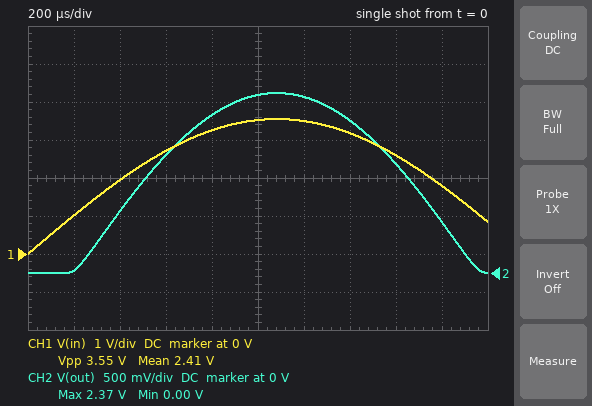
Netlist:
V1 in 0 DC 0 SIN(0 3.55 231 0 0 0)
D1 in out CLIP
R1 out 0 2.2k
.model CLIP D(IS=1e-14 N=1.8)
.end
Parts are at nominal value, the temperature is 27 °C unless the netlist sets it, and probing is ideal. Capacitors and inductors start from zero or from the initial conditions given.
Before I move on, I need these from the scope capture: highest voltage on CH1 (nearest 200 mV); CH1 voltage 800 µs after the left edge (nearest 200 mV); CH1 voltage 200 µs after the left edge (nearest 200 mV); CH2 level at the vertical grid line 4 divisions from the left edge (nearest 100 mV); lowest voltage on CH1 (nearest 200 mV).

3.6 V
3.2 V
1.0 V
2.1 V
0 V
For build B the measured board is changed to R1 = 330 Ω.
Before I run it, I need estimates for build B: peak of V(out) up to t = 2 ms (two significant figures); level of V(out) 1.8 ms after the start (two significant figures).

2.3 V
590 mV
